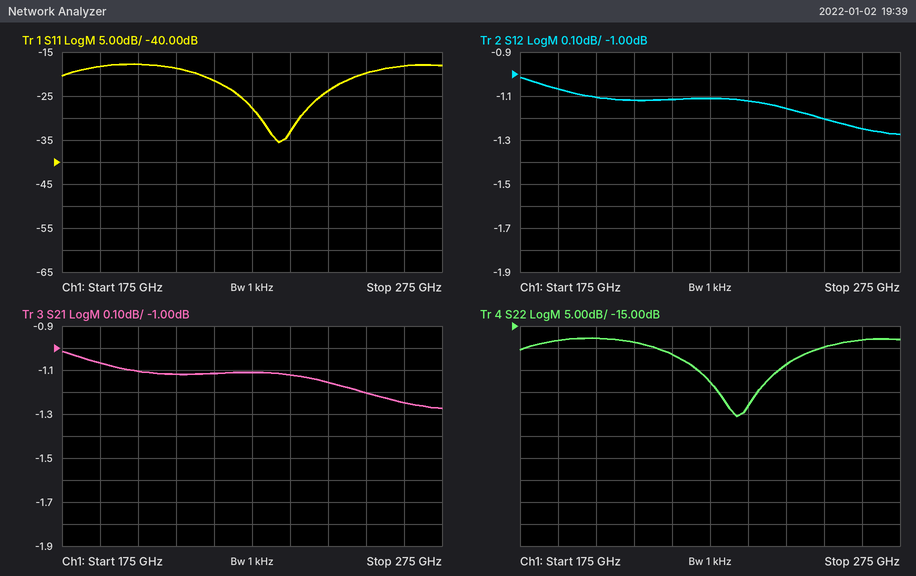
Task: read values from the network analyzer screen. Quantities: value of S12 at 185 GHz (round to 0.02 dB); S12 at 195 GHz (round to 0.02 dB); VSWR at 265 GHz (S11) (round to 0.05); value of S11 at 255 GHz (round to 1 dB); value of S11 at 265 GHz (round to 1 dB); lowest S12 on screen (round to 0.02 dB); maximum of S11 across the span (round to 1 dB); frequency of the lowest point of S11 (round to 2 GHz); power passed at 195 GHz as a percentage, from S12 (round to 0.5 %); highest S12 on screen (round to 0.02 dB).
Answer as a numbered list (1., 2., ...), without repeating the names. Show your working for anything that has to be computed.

1. -1.06 dB
2. -1.10 dB
3. |Γ| = 10^(-18/20) = 0.1259; VSWR = (1 + 0.1259)/(1 − 0.1259) ≈ 1.29, so 1.30 to the nearest 0.05
4. -20 dB
5. -18 dB
6. -1.28 dB
7. -18 dB
8. 232 GHz
9. 10^(-1.1/10) ≈ 77.6 %, so 77.5 % to the nearest 0.5 %
10. -1.02 dB
